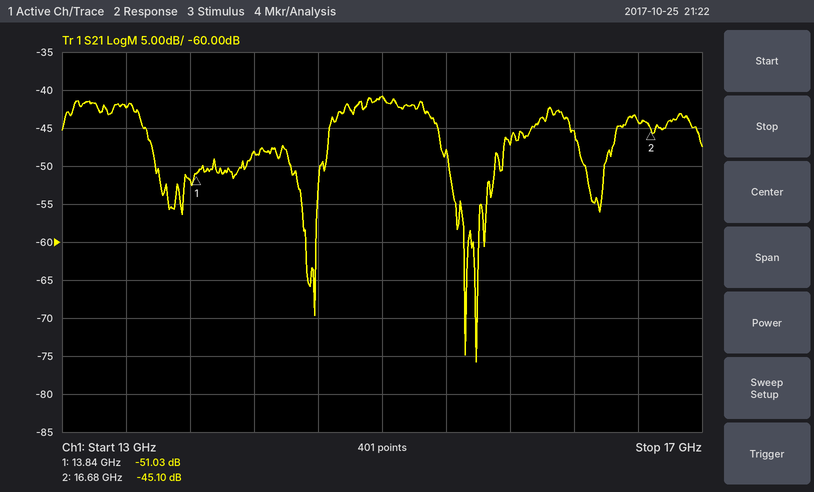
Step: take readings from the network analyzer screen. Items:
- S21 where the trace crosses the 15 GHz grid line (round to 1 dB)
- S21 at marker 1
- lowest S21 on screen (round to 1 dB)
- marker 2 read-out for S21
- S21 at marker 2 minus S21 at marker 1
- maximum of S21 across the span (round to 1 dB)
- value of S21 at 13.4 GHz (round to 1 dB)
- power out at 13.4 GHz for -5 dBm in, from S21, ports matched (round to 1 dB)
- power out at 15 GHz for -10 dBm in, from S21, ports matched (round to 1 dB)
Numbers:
-41 dB
-51.03 dB
-76 dB
-45.10 dB
5.93 dB
-41 dB
-42 dB
-47 dBm
-51 dBm
